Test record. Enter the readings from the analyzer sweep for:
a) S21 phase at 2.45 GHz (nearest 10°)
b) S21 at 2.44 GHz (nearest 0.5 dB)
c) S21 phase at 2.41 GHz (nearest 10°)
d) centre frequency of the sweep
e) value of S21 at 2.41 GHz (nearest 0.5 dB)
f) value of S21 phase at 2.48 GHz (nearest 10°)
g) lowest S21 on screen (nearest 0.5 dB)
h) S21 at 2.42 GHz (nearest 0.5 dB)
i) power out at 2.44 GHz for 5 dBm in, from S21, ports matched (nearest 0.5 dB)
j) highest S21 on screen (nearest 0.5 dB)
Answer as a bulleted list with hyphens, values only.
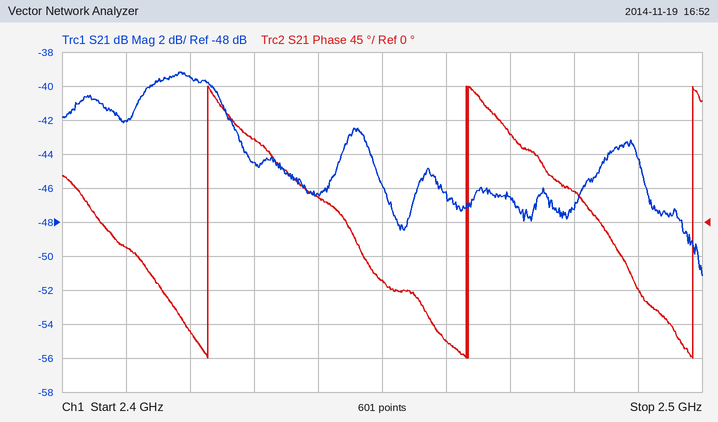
- -80°
- -46.5 dB
- -30°
- 2.45 GHz
- -42.0 dB
- 40°
- -51.0 dB
- -39.5 dB
- -41.5 dBm
- -39.0 dB
